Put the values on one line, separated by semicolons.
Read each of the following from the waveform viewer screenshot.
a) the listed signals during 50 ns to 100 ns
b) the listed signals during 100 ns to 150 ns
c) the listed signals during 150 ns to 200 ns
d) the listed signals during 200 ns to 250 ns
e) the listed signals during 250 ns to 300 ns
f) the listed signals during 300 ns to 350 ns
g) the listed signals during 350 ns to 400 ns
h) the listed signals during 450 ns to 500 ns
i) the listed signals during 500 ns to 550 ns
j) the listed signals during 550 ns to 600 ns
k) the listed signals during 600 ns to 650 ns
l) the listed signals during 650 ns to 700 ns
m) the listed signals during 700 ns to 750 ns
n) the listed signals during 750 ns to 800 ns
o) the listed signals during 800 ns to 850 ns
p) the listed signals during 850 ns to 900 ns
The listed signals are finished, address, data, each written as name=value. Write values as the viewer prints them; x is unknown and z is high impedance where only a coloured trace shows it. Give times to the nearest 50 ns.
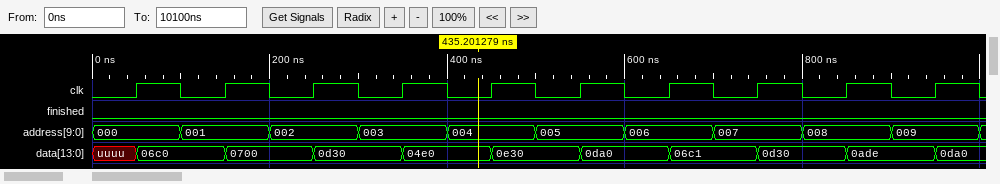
finished=0, address=000, data=06c0; finished=0, address=001, data=06c0; finished=0, address=001, data=0700; finished=0, address=002, data=0700; finished=0, address=002, data=0d30; finished=0, address=003, data=0d30; finished=0, address=003, data=04e0; finished=0, address=004, data=0e30; finished=0, address=005, data=0e30; finished=0, address=005, data=0da0; finished=0, address=006, data=0da0; finished=0, address=006, data=06c1; finished=0, address=007, data=06c1; finished=0, address=007, data=0d30; finished=0, address=008, data=0d30; finished=0, address=008, data=0ade
